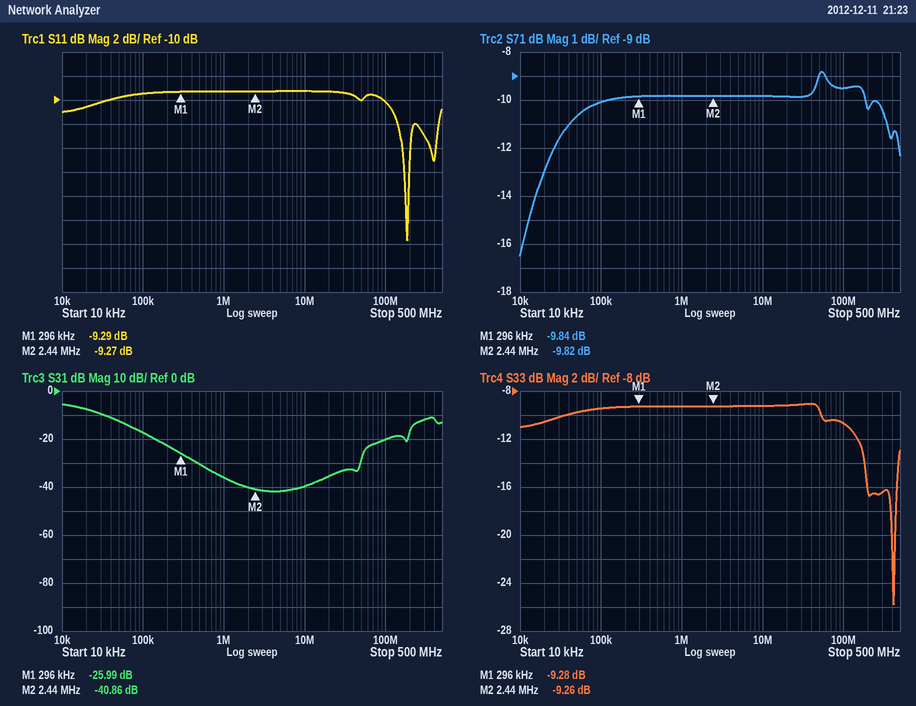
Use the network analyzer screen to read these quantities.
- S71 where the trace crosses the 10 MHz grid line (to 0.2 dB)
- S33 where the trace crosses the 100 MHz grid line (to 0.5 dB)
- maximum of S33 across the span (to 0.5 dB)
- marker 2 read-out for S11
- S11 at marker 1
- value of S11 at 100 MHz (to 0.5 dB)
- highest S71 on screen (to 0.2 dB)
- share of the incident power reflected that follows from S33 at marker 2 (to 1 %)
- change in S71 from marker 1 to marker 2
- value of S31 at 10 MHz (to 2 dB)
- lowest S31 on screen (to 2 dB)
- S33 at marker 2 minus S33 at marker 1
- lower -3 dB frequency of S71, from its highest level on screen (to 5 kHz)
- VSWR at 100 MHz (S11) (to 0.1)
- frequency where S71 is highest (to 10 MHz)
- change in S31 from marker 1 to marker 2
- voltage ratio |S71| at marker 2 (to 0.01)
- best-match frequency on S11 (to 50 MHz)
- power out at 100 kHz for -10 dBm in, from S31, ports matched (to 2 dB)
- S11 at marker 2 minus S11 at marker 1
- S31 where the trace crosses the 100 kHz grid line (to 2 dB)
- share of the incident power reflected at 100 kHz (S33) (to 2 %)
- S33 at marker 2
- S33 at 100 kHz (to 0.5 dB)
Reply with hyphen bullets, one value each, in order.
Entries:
- -9.8 dB
- -10.5 dB
- -9.0 dB
- -9.27 dB
- -9.29 dB
- -10.0 dB
- -8.8 dB
- 12 %
- 0.02 dB
- -40 dB
- -42 dB
- 0.02 dB
- 30 kHz
- 1.9
- 50 MHz
- -14.87 dB
- 0.32
- 200 MHz
- -28 dBm
- 0.02 dB
- -18 dB
- 12 %
- -9.26 dB
- -9.5 dB
